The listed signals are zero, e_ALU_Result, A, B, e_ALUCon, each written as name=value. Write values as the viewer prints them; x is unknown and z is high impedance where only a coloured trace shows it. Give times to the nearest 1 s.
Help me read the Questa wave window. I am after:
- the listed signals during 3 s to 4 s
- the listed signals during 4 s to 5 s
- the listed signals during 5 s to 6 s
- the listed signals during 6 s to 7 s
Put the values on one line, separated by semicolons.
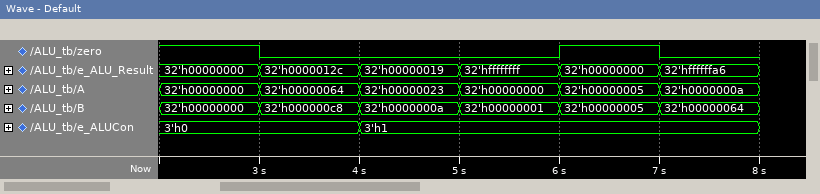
zero=0, e_ALU_Result=32'h0000012c, A=32'h00000064, B=32'h000000c8, e_ALUCon=3'h0; zero=0, e_ALU_Result=32'h00000019, A=32'h00000023, B=32'h0000000a, e_ALUCon=3'h1; zero=0, e_ALU_Result=32'hffffffff, A=32'h00000000, B=32'h00000001, e_ALUCon=3'h1; zero=1, e_ALU_Result=32'h00000000, A=32'h00000005, B=32'h00000005, e_ALUCon=3'h1
